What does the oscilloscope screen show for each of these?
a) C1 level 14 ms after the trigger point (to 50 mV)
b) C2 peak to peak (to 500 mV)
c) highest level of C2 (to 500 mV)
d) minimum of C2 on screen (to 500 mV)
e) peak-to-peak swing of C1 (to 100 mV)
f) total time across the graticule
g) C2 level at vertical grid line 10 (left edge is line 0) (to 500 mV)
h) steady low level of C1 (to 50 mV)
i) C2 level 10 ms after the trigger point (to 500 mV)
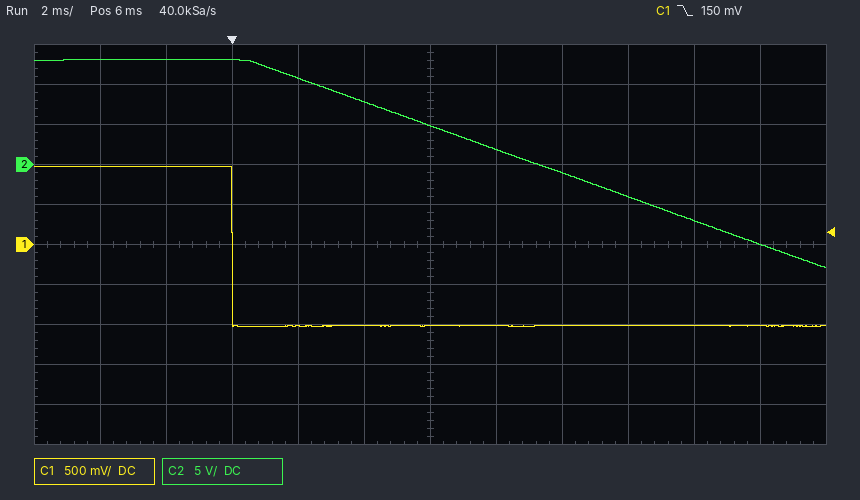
-1.00 V
26.0 V
13.0 V
-13.0 V
2.00 V
24 ms
-7.0 V
-1.00 V
-1.0 V
